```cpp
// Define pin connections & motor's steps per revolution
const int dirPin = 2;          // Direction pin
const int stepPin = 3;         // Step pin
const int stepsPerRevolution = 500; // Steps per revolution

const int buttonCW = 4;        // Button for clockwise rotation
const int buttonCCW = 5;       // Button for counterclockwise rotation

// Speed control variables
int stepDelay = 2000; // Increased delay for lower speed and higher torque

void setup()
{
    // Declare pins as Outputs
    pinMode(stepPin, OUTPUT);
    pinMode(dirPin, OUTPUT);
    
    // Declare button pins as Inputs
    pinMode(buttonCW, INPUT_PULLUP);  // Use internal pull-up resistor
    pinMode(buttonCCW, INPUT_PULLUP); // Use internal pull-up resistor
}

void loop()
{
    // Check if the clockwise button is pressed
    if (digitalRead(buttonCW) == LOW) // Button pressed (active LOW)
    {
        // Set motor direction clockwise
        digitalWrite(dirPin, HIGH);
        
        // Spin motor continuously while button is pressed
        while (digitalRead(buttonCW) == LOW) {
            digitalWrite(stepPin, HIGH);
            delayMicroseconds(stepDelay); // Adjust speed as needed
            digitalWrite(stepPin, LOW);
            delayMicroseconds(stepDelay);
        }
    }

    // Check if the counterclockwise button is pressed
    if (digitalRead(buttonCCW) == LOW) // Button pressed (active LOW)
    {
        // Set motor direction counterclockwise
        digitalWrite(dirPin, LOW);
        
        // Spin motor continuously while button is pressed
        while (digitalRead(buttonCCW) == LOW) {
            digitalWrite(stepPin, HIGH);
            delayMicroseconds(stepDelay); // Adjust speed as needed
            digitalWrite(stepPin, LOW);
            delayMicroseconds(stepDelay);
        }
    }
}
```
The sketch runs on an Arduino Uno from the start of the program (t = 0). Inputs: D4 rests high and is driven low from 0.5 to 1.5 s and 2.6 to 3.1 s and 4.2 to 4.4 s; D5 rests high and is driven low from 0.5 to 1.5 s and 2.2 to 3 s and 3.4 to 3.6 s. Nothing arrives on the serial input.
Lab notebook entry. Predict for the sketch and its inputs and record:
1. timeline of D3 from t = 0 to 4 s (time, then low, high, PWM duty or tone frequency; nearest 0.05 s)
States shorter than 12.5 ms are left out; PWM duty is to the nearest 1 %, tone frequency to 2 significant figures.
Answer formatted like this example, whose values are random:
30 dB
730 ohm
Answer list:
0 s low; 0.5 s tone 250 Hz; 1.5 s low; 2.2 s tone 250 Hz; 3.1 s low; 3.4 s tone 250 Hz; 3.6 s low
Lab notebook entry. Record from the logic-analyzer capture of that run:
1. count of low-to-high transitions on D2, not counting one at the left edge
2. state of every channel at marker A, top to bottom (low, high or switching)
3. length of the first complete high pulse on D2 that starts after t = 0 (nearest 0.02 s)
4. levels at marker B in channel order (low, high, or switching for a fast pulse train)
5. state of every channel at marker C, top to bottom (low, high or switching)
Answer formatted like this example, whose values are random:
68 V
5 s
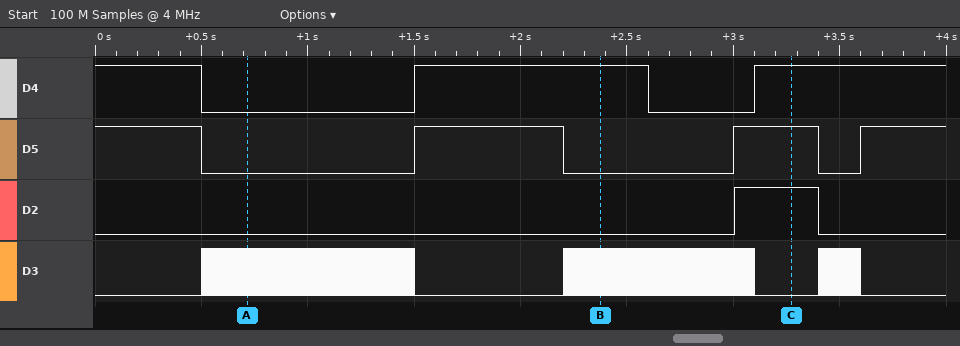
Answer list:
1
D4 low, D5 low, D2 low, D3 switching
0.40 s
D4 high, D5 low, D2 low, D3 switching
D4 high, D5 high, D2 high, D3 low
